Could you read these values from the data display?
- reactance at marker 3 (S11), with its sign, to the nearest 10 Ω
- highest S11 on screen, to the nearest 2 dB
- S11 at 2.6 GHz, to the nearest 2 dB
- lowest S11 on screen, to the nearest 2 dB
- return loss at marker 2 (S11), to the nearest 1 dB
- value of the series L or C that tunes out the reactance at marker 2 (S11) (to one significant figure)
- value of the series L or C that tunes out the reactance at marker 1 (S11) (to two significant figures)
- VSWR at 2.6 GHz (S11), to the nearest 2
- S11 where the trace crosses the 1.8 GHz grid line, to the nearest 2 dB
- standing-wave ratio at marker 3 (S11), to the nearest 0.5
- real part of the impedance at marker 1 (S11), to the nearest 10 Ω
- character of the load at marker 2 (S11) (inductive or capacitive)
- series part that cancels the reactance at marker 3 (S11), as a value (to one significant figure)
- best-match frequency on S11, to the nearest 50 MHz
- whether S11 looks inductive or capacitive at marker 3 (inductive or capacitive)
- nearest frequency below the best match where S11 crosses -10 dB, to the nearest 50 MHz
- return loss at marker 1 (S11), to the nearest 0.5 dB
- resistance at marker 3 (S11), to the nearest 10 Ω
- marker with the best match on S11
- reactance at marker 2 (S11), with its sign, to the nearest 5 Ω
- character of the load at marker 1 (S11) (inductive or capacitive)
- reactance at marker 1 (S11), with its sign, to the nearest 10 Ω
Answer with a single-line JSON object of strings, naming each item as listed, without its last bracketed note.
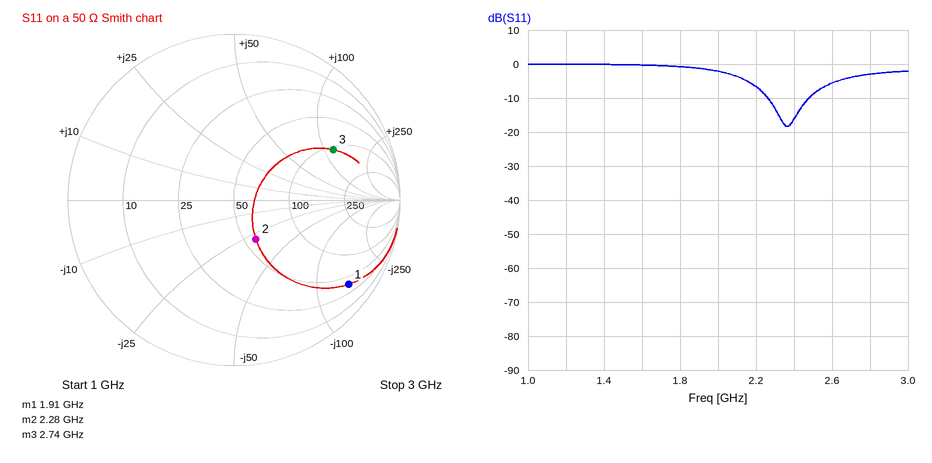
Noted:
{"reactance at marker 3 (S11), with its sign, to the nearest 10 Ω": "+120 Ω", "highest S11 on screen, to the nearest 2 dB": "0 dB", "S11 at 2.6 GHz, to the nearest 2 dB": "-6 dB", "lowest S11 on screen, to the nearest 2 dB": "-18 dB", "return loss at marker 2 (S11), to the nearest 1 dB": "11 dB", "value of the series L or C that tunes out the reactance at marker 2 (S11)": "2 nH", "value of the series L or C that tunes out the reactance at marker 1 (S11)": "12 nH", "VSWR at 2.6 GHz (S11), to the nearest 2": "4", "S11 where the trace crosses the 1.8 GHz grid line, to the nearest 2 dB": "0 dB", "standing-wave ratio at marker 3 (S11), to the nearest 0.5": "5.0", "real part of the impedance at marker 1 (S11), to the nearest 10 Ω": "40 Ω", "character of the load at marker 2 (S11)": "capacitive", "series part that cancels the reactance at marker 3 (S11), as a value": "500 fF", "best-match frequency on S11, to the nearest 50 MHz": "2.35 GHz", "whether S11 looks inductive or capacitive at marker 3": "inductive", "nearest frequency below the best match where S11 crosses -10 dB, to the nearest 50 MHz": "2.25 GHz", "return loss at marker 1 (S11), to the nearest 0.5 dB": "1.5 dB", "resistance at marker 3 (S11), to the nearest 10 Ω": "110 Ω", "marker with the best match on S11": "marker 2", "reactance at marker 2 (S11), with its sign, to the nearest 5 Ω": "-30 Ω", "character of the load at marker 1 (S11)": "capacitive", "reactance at marker 1 (S11), with its sign, to the nearest 10 Ω": "-140 Ω"}
